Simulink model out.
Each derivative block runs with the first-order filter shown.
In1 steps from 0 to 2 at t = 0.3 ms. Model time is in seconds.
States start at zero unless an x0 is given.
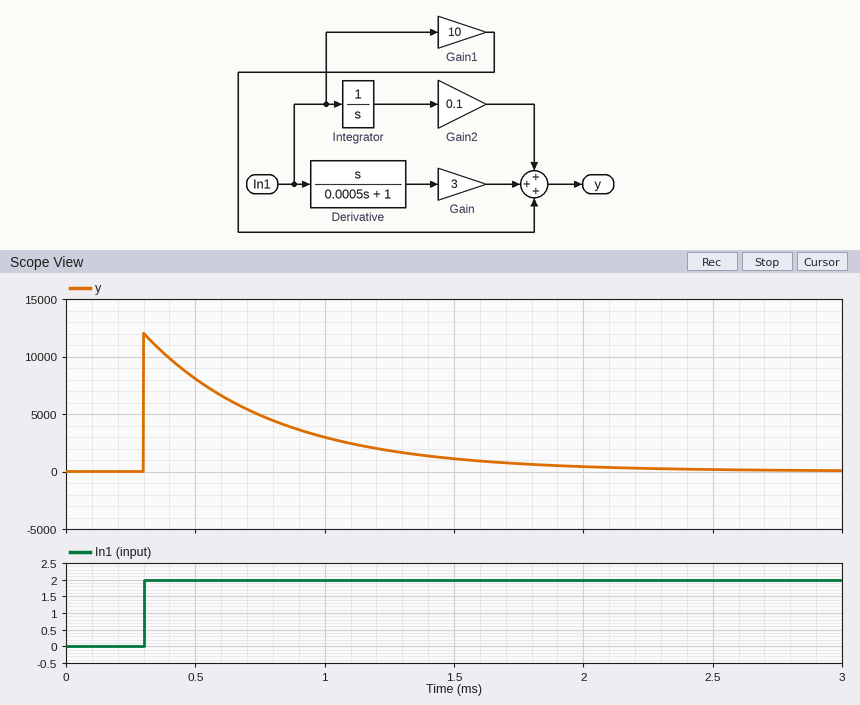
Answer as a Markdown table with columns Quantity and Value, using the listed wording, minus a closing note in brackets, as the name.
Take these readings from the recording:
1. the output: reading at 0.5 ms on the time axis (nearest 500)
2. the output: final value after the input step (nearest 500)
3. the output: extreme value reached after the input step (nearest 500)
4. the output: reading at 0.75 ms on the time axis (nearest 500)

| Quantity | Value |
|---|---|
| the output: reading at 0.5 ms on the time axis | 8000 |
| the output: final value after the input step | 0 |
| the output: extreme value reached after the input step | 12000 |
| the output: reading at 0.75 ms on the time axis | 5000 |
